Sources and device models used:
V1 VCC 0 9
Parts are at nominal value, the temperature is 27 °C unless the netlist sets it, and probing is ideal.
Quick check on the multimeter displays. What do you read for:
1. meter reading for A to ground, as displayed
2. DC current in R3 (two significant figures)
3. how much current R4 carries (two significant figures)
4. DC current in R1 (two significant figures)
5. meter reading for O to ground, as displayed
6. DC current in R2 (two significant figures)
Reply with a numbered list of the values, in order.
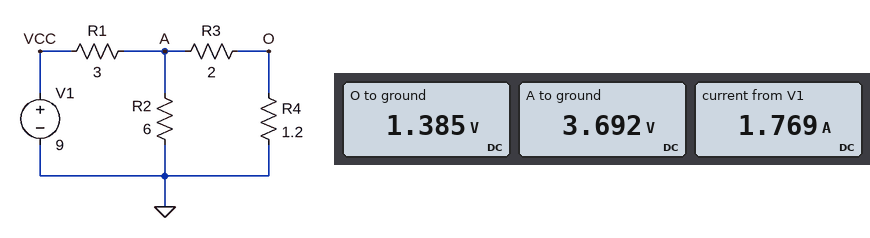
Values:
1. 3.692 V
2. 1.2 A
3. 1.2 A
4. 1.8 A
5. 1.385 V
6. 620 mA
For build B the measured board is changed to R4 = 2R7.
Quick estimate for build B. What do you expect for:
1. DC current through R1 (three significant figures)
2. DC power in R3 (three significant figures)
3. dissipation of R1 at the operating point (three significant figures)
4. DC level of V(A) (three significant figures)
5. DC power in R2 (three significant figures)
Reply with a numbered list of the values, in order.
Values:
1. 1.60 A
2. 1.60 W
3. 7.65 W
4. 4.21 V
5. 2.95 W
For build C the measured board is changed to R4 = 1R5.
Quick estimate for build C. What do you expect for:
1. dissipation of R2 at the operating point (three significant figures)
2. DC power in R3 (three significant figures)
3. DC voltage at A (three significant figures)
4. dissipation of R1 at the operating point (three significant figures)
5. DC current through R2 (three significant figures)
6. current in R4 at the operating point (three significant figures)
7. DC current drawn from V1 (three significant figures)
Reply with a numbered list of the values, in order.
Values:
1. 2.43 W
2. 2.38 W
3. 3.82 V
4. 8.95 W
5. 636 mA
6. 1.09 A
7. 1.73 A
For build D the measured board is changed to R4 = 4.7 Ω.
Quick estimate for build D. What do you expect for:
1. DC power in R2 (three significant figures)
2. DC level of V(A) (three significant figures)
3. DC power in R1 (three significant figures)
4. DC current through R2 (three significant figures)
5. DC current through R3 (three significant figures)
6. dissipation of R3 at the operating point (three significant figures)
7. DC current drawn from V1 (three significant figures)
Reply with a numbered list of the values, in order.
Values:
1. 3.56 W
2. 4.62 V
3. 6.39 W
4. 770 mA
5. 690 mA
6. 951 mW
7. 1.46 A
